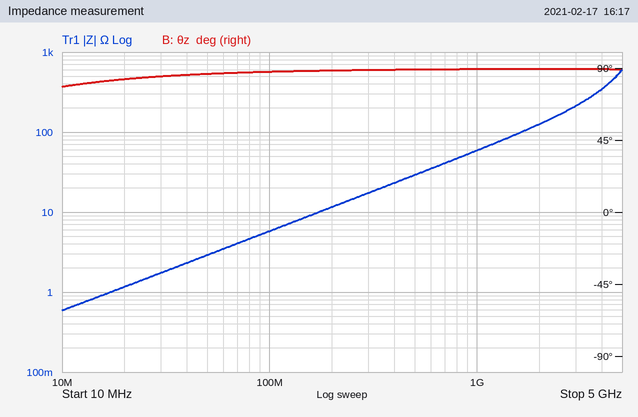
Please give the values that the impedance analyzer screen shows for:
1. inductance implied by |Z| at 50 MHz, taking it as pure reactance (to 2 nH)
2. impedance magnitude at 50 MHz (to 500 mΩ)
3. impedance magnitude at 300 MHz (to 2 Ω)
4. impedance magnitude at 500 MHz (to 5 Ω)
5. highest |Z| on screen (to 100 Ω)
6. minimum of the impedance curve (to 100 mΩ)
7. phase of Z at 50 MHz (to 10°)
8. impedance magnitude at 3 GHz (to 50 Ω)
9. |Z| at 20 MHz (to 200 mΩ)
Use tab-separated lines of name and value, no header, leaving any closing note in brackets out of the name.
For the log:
inductance implied by |Z| at 50 MHz, taking it as pure reactance	10 nH
impedance magnitude at 50 MHz	3.0 Ω
impedance magnitude at 300 MHz	18 Ω
impedance magnitude at 500 MHz	30 Ω
highest |Z| on screen	600 Ω
minimum of the impedance curve	600 mΩ
phase of Z at 50 MHz	90°
impedance magnitude at 3 GHz	200 Ω
|Z| at 20 MHz	1.2 Ω
